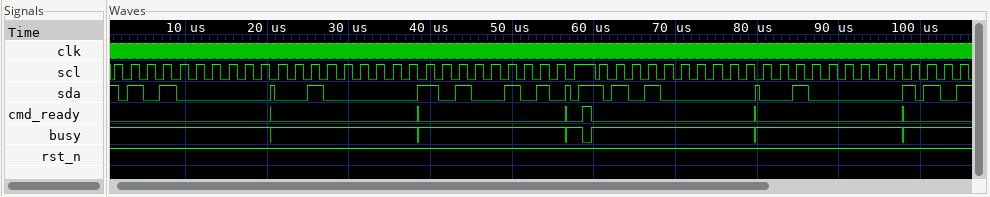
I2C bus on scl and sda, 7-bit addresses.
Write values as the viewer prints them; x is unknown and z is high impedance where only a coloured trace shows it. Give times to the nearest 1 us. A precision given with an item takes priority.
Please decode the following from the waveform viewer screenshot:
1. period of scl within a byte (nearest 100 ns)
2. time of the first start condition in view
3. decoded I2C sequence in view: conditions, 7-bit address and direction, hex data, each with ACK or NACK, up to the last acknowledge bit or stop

2000 ns
2 us
start, address 50 write ACK, 20 ACK, A5 ACK, stop, start, address 50 write ACK, 20 ACK
